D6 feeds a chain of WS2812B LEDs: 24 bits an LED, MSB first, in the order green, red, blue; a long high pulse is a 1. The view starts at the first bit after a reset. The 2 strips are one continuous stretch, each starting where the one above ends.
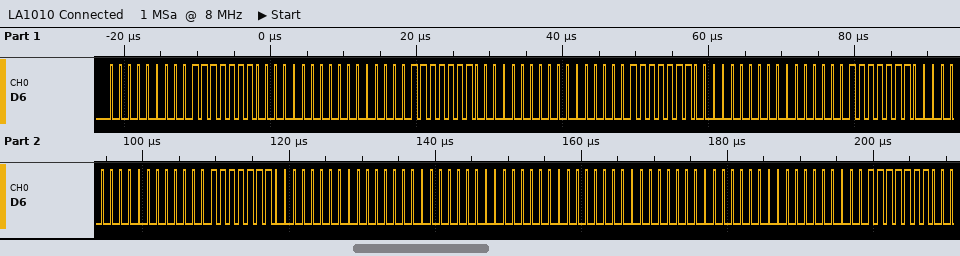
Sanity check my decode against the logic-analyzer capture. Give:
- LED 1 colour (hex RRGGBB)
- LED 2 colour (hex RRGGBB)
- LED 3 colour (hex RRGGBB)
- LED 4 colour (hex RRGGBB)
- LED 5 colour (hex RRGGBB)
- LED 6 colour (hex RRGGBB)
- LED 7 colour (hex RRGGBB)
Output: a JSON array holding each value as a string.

["#7F0000", "#7F0000", "#7F0000", "#7F0000", "#7F0000", "#000000", "#000000"]
